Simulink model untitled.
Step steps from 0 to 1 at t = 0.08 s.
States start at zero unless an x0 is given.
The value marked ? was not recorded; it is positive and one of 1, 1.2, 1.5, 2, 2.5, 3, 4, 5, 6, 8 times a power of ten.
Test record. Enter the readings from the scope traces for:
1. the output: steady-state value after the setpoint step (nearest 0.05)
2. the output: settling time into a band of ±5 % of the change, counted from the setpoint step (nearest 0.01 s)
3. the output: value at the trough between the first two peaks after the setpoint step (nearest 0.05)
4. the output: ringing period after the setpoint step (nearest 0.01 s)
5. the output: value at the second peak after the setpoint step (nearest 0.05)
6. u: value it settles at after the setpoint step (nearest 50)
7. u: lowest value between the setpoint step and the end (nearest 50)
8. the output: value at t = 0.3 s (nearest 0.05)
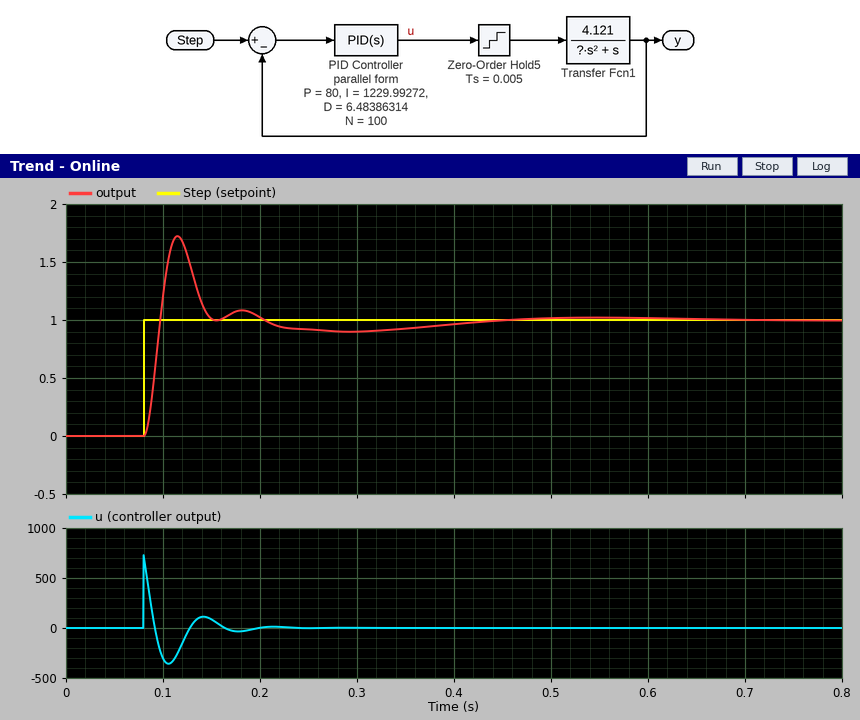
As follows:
1.00
0.30 s
1.00
0.07 s
1.10
0
-350
0.90
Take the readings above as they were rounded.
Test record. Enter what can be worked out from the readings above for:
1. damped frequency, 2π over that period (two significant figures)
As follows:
90 rad/s
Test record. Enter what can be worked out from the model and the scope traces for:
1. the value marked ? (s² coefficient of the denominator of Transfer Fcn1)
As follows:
0.3
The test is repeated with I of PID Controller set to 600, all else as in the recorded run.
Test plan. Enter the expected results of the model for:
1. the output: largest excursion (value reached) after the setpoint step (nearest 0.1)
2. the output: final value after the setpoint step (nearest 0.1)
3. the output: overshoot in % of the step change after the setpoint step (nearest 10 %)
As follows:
1.7
1.0
70 %
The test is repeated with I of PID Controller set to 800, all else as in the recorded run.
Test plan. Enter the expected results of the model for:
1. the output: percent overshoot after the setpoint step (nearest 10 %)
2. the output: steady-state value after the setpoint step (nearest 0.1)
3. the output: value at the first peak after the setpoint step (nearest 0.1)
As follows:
70 %
1.0
1.7
